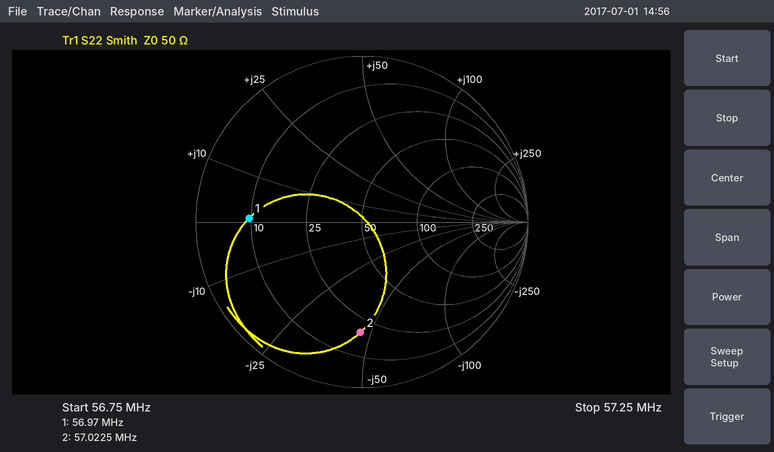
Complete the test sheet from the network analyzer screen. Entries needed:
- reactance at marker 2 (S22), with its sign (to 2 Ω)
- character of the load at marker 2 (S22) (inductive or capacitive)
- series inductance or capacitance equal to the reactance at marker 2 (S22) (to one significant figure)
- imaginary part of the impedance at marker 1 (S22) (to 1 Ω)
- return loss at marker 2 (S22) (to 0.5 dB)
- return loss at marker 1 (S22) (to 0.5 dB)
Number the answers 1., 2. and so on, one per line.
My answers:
1. -46 Ω
2. capacitive
3. 60 pF
4. +1 Ω
5. 3.5 dB
6. 3.5 dB
